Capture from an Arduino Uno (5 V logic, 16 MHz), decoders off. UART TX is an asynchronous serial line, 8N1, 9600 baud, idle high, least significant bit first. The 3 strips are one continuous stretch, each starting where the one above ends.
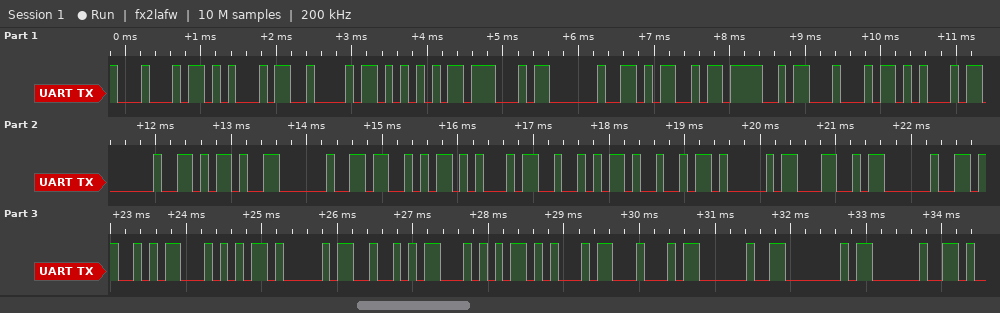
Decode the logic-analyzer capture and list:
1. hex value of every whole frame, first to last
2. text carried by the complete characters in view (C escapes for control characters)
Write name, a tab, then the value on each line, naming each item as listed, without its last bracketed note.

hex value of every whole frame, first to last	44 45 42 55 47 20 4D 4F 44 45 20 2D 20 53 45 52 49 41 4C 20 53 54 41 52 54 45 44 20 40 20
text carried by the complete characters in view	"DEBUG MODE - SERIAL STARTED @ "
